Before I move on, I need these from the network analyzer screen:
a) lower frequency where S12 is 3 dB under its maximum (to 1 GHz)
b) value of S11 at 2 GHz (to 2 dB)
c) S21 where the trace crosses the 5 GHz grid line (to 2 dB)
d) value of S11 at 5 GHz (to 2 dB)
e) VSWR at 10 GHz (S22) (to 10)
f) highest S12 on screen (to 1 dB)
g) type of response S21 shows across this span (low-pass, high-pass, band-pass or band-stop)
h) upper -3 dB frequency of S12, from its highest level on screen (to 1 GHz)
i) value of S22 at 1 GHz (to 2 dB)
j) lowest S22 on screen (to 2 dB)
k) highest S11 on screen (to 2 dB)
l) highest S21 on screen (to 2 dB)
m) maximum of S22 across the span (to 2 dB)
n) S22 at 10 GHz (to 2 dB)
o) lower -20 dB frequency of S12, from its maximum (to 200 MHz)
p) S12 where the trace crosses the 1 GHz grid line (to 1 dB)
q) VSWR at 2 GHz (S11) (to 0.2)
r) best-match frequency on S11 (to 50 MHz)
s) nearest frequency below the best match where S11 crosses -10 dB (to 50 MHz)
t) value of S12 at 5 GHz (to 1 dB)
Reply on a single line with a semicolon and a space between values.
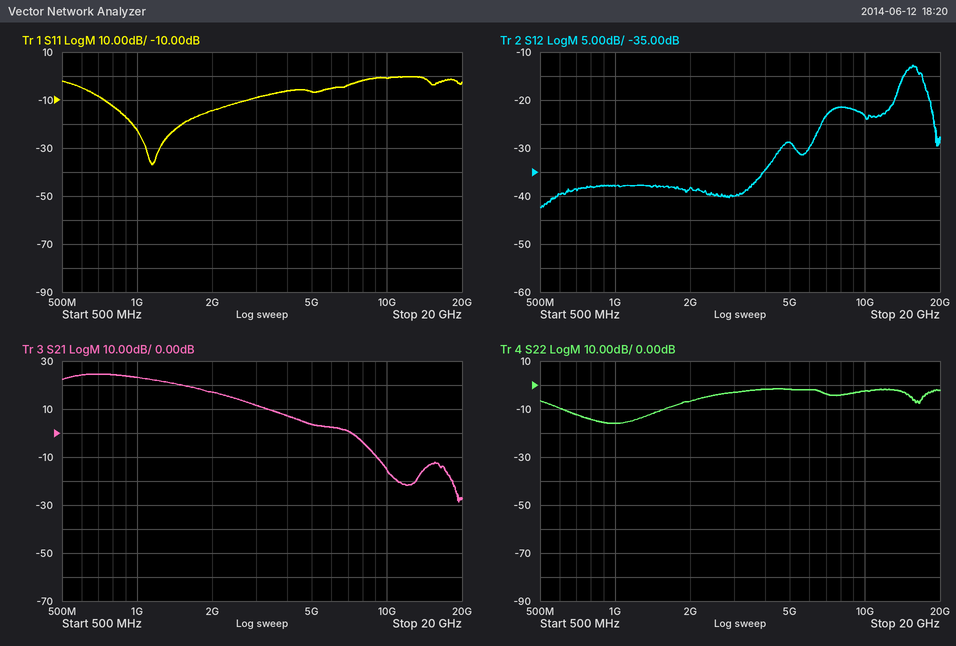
14 GHz; -14 dB; 4 dB; -6 dB; 10; -13 dB; low-pass; 17 GHz; -16 dB; -16 dB; 0 dB; 24 dB; -2 dB; -2 dB; 4.2 GHz; -38 dB; 1.4; 1.15 GHz; 750 MHz; -29 dB
